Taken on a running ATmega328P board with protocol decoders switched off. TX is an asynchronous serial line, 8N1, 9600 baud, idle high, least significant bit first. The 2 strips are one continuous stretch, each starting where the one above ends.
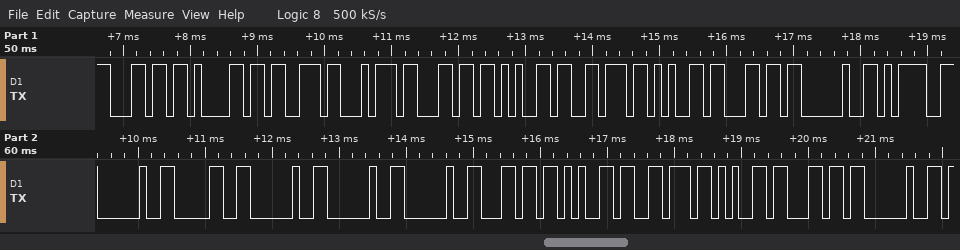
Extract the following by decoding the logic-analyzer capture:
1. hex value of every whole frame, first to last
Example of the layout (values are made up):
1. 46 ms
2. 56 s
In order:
1. 0x6C 0x61 0x73 0x74 0x6C 0x65 0x76 0x65 0x6C 0x20 0x3D 0x20 0x30 0x20 0x20 0x20 0x6C 0x65 0x76 0x65 0x6C 0x20
